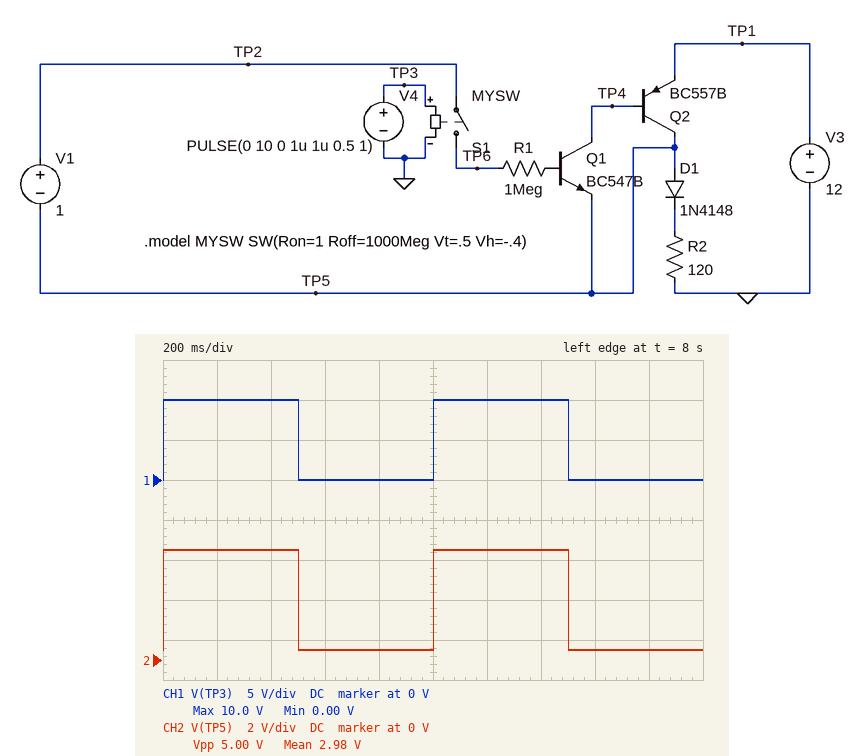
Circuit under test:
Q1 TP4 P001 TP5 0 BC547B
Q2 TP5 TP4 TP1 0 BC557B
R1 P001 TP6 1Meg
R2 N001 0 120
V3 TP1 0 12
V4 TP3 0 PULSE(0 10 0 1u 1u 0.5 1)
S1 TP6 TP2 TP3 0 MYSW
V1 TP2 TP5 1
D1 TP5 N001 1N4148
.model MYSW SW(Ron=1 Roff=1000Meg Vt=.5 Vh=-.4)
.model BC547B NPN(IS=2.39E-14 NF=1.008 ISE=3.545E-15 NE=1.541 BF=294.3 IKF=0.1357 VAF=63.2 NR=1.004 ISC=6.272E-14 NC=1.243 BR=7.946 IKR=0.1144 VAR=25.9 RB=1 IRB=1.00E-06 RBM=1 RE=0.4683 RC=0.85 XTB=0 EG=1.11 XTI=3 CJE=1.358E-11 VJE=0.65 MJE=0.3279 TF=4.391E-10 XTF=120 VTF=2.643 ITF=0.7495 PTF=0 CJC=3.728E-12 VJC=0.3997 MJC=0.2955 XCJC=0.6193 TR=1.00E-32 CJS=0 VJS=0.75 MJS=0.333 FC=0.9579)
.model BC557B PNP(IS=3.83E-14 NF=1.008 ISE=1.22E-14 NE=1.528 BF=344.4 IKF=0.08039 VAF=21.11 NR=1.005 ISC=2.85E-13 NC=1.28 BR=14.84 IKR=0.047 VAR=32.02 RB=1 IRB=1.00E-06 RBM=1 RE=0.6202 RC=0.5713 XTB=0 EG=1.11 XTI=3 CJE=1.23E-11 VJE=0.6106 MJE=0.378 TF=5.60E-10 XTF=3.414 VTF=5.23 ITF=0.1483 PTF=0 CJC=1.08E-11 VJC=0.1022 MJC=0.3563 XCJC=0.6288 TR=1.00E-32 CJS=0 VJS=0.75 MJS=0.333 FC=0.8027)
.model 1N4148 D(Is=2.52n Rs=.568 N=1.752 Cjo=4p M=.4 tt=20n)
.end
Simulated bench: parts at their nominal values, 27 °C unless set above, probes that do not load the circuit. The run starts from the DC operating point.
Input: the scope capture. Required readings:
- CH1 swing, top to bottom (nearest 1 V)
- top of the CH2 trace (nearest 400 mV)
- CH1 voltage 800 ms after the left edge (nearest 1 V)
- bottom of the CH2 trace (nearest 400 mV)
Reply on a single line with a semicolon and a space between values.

10 V; 5.6 V; 0 V; 400 mV
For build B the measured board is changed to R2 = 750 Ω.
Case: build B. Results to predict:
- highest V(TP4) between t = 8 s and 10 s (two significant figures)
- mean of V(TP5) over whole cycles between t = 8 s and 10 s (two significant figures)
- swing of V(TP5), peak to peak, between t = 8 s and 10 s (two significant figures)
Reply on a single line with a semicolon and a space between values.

11 V; 5.9 V; 11 V
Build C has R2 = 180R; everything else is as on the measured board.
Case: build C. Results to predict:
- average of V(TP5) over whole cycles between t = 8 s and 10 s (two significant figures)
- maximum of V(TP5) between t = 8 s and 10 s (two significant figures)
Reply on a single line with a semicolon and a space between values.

3.9 V; 7.2 V
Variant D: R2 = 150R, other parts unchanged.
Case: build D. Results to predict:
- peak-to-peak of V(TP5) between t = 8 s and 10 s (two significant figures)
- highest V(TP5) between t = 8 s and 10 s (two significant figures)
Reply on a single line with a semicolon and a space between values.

5.9 V; 6.4 V
